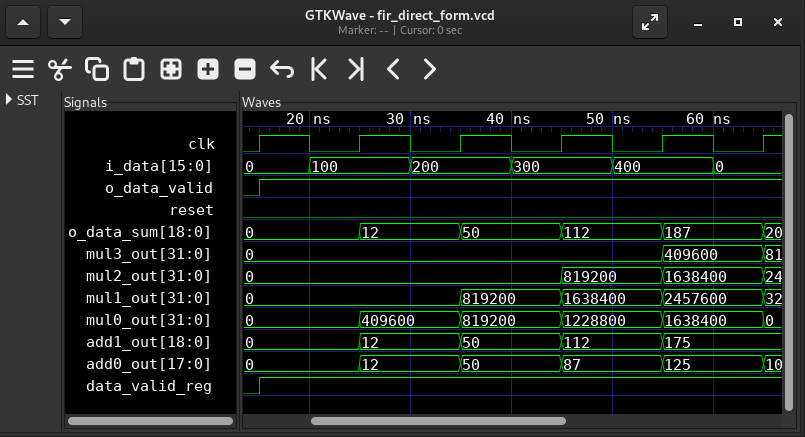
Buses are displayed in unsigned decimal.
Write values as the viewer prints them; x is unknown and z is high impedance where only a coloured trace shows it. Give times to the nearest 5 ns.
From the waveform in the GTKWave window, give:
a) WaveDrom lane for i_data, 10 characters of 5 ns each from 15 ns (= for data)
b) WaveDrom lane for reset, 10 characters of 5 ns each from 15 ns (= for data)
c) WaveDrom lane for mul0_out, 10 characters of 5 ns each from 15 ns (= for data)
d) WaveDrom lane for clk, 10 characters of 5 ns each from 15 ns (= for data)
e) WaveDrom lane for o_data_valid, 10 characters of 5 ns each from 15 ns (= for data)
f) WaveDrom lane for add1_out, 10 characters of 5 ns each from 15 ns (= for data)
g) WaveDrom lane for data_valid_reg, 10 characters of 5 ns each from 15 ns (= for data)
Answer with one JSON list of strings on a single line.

["{name: 'i_data', wave: '==.=.=.=.=', data: '0 100 200 300 400 0'}", "{name: 'reset', wave: '0.........'}", "{name: 'mul0_out', wave: '=.=.=.=.=.', data: '0 409600 819200 1228800 1638400'}", "{name: 'clk', wave: '1010101010'}", "{name: 'o_data_valid', wave: '1.........'}", "{name: 'add1_out', wave: '=.=.=.=.=.', data: '0 12 50 112 175'}", "{name: 'data_valid_reg', wave: '1.........'}"]
